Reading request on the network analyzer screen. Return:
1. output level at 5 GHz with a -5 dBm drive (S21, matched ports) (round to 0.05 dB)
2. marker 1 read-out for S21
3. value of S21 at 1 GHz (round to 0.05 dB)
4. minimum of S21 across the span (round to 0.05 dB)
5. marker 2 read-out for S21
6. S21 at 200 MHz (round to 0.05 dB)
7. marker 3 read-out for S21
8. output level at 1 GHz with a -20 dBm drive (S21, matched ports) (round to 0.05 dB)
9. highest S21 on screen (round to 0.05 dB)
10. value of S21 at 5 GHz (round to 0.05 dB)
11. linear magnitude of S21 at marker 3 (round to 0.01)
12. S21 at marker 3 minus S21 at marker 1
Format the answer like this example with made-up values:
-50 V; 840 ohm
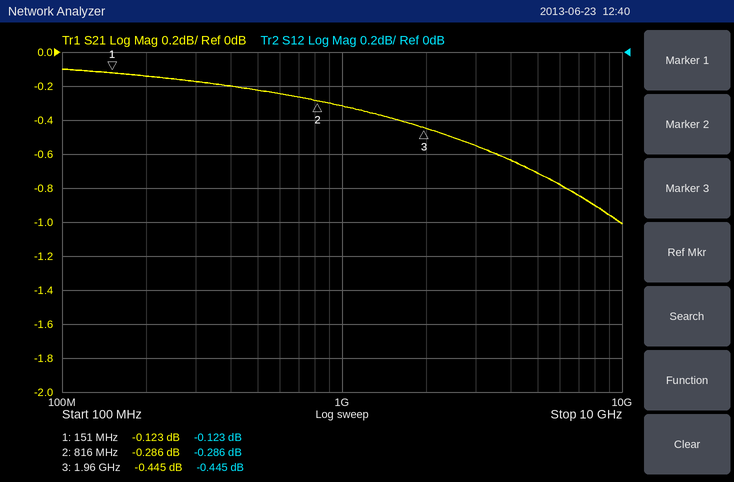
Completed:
-5.70 dBm; -0.123 dB; -0.30 dB; -1.00 dB; -0.286 dB; -0.15 dB; -0.445 dB; -20.30 dBm; -0.10 dB; -0.70 dB; 0.95; -0.322 dB
